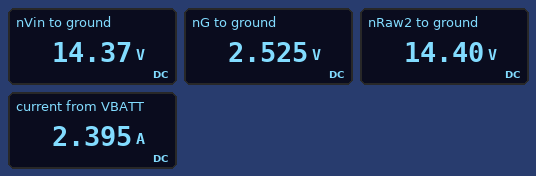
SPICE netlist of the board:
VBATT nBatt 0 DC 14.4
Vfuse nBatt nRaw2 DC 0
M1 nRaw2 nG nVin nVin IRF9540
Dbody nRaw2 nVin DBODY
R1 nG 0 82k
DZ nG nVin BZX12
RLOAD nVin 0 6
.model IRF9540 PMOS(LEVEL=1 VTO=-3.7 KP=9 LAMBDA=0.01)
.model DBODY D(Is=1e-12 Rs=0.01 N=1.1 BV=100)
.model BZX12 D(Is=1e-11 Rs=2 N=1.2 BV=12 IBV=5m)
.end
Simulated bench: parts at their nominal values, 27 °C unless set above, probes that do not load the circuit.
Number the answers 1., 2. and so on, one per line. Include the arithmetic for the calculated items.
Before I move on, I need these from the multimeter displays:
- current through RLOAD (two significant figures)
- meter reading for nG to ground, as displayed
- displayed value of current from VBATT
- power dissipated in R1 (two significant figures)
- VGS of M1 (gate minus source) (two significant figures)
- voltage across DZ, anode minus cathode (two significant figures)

1. (14.37 V) / 6 Ω = 2.4 A
2. 2.525 V
3. 2.395 A
4. (2.525 V)^2 / 82 kΩ = 78 µW
5. 2.525 V - 14.37 V = -12 V
6. 2.525 V - 14.37 V = -12 V
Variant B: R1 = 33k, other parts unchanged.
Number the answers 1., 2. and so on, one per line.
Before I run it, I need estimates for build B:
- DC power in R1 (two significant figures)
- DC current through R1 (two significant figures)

1. 190 µW
2. 76 µA
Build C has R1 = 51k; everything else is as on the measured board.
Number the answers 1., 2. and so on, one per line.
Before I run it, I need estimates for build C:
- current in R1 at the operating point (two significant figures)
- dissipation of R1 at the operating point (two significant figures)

1. 49 µA
2. 120 µW
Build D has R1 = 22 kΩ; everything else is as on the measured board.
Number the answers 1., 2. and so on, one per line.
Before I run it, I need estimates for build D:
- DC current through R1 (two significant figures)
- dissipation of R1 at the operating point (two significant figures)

1. 110 µA
2. 280 µW
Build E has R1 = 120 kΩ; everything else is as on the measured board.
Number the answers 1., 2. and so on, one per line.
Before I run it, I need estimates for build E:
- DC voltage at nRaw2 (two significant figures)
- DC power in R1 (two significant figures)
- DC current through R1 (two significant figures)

1. 14 V
2. 54 µW
3. 21 µA
